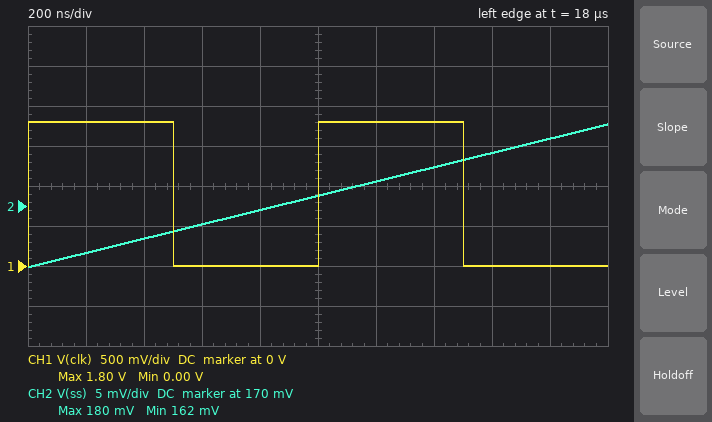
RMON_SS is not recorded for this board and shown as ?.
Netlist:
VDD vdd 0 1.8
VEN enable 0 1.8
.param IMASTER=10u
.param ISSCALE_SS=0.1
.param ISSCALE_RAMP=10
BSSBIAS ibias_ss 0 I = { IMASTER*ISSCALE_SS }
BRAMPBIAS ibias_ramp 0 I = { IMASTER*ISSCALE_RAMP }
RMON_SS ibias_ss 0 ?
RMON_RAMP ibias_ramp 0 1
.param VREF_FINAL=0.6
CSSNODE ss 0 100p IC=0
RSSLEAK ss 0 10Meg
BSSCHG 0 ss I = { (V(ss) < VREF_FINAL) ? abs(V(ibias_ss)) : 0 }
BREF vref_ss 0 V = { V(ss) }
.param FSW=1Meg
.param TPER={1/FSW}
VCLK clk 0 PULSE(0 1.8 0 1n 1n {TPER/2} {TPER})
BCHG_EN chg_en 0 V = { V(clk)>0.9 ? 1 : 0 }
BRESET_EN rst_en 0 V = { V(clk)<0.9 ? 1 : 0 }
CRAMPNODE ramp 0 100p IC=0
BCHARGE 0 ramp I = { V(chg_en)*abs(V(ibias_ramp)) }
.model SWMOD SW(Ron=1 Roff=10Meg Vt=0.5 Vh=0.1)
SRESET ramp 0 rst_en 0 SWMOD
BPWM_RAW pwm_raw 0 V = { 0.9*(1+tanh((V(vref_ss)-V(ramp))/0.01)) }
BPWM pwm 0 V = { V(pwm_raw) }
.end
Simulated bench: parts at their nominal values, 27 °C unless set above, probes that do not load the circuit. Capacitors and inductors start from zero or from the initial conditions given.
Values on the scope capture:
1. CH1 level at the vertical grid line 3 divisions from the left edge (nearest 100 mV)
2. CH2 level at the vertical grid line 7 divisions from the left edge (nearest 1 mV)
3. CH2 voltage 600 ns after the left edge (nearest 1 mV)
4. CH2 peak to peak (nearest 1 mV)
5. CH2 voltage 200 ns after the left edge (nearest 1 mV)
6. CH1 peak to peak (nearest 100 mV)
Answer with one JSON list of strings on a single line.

["0 V", "175 mV", "168 mV", "18 mV", "164 mV", "1.8 V"]
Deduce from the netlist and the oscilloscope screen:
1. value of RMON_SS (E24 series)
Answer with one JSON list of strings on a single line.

["0.91 Ω"]
